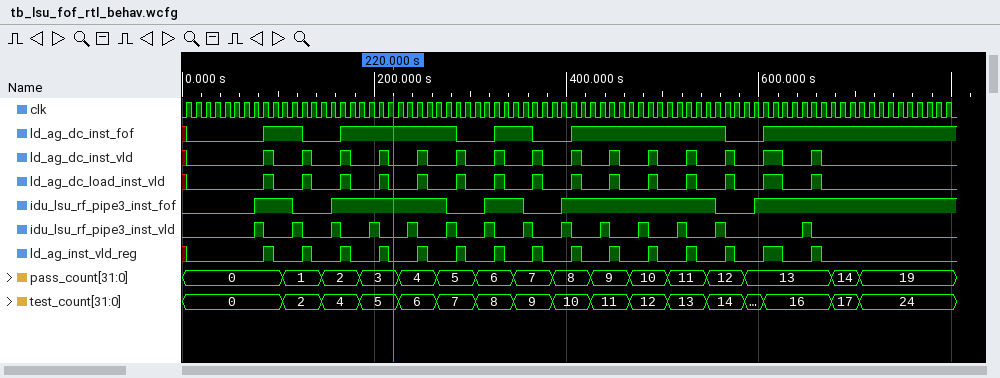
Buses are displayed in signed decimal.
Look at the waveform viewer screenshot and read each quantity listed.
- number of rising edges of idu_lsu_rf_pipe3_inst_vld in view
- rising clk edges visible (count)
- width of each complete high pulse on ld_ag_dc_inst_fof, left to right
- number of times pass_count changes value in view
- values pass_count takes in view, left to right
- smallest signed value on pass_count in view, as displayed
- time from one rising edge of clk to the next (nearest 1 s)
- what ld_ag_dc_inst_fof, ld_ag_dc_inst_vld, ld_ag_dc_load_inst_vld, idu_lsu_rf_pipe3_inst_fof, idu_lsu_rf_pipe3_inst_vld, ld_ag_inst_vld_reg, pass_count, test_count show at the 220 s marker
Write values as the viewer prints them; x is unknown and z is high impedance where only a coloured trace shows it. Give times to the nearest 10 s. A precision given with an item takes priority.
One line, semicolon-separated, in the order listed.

14; 80; 40 s, 120 s, 40 s, 160 s; 15; 0, 1, 2, 3, 4, 5, 6, 7, 8, 9, 10, 11, 12, 13, 14, 19; 0; 10 s; ld_ag_dc_inst_fof=1, ld_ag_dc_inst_vld=0, ld_ag_dc_load_inst_vld=0, idu_lsu_rf_pipe3_inst_fof=1, idu_lsu_rf_pipe3_inst_vld=0, ld_ag_inst_vld_reg=0, pass_count=3, test_count=5
